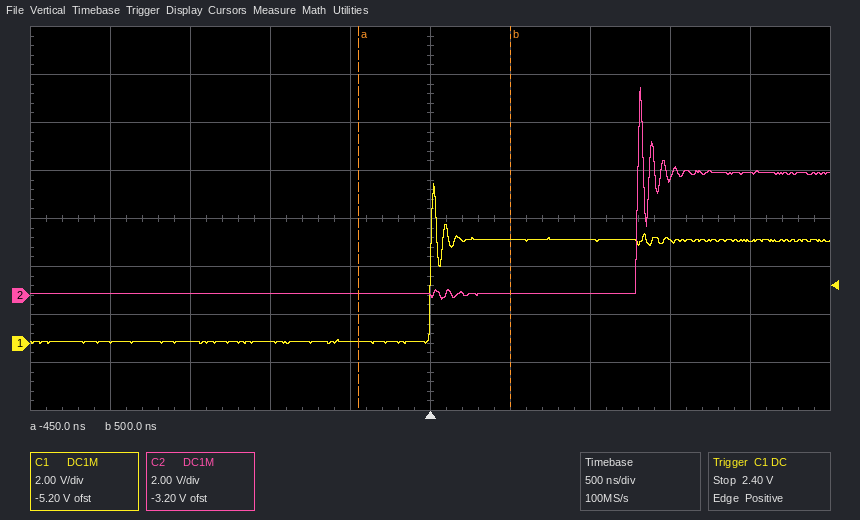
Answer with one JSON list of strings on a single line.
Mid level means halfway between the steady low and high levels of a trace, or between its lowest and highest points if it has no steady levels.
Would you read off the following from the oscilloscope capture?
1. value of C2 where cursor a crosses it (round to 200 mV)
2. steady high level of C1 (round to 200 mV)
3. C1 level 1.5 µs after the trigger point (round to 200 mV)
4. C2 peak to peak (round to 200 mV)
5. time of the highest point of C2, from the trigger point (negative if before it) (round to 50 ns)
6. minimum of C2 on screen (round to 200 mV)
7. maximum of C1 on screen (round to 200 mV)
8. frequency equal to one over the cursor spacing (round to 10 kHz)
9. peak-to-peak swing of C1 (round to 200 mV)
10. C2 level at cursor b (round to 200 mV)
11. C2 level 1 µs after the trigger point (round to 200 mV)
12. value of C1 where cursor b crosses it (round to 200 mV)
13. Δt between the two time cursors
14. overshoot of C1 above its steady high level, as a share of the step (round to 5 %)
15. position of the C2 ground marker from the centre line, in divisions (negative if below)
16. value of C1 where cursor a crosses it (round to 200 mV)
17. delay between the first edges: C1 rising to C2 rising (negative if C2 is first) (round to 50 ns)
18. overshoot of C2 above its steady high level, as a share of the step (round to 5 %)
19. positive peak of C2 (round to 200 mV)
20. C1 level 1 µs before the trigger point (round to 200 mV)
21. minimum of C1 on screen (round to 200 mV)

["0.0 V", "4.4 V", "4.2 V", "8.8 V", "+1.30 µs", "-200 mV", "6.6 V", "1.05 MHz", "6.6 V", "0.0 V", "0.0 V", "4.4 V", "950 ns", "55 %", "-1.6 div", "0.0 V", "+1.30 µs", "70 %", "8.6 V", "0.0 V", "0.0 V"]
